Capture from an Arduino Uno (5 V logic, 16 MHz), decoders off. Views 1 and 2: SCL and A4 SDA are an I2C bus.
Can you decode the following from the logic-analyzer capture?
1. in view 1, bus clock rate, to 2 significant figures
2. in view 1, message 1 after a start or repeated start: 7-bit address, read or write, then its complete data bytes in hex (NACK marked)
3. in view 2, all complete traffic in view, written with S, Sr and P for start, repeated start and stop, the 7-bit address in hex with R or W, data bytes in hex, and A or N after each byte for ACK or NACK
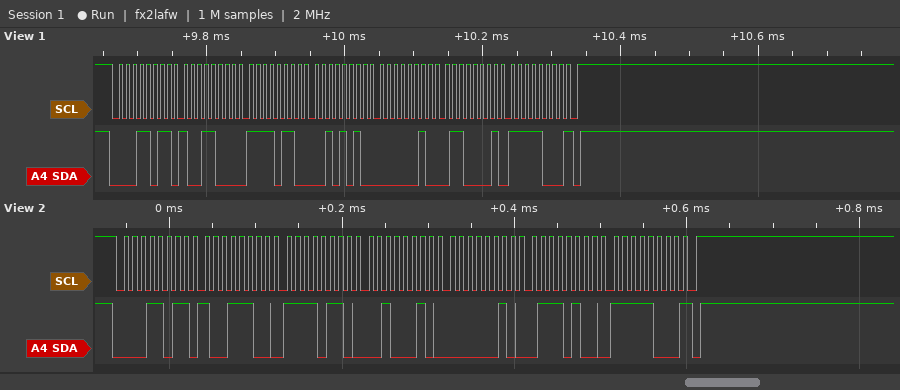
100 kHz
0x0D read: 98 F6 2A 02 61 F8 NACK
S 0DR A 9C A F6 A 22 A 02 A 74 A F8 N P
